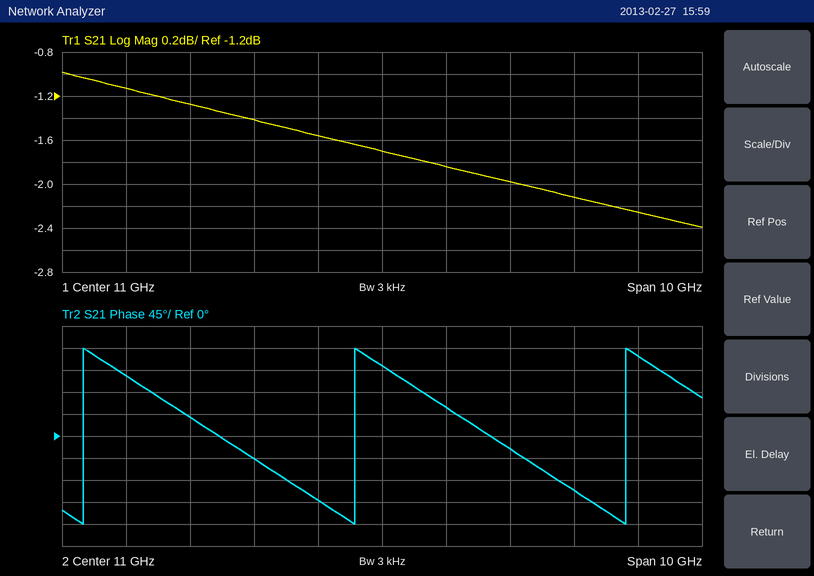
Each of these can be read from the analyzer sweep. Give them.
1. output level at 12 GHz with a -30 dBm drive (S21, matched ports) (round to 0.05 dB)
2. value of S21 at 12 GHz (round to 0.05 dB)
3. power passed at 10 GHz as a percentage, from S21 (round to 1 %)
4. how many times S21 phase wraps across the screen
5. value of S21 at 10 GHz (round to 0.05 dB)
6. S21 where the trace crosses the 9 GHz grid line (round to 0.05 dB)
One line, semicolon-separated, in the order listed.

-31.85 dBm; -1.85 dB; 70 %; 3; -1.55 dB; -1.40 dB
